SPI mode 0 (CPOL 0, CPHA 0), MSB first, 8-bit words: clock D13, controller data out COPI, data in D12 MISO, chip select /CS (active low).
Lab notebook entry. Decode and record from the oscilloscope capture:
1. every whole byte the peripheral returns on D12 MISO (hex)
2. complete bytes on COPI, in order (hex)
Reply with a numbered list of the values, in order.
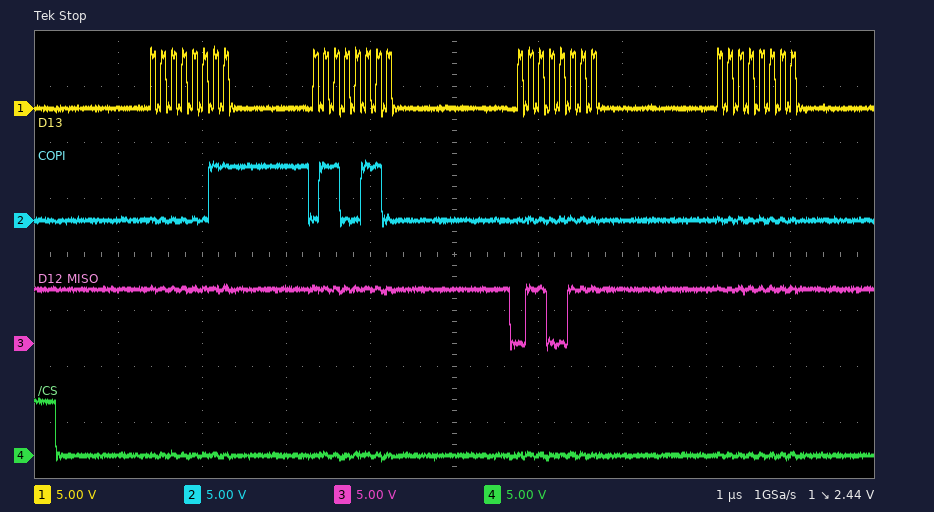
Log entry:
1. FF FF 67 FF
2. 03 66 00 00
